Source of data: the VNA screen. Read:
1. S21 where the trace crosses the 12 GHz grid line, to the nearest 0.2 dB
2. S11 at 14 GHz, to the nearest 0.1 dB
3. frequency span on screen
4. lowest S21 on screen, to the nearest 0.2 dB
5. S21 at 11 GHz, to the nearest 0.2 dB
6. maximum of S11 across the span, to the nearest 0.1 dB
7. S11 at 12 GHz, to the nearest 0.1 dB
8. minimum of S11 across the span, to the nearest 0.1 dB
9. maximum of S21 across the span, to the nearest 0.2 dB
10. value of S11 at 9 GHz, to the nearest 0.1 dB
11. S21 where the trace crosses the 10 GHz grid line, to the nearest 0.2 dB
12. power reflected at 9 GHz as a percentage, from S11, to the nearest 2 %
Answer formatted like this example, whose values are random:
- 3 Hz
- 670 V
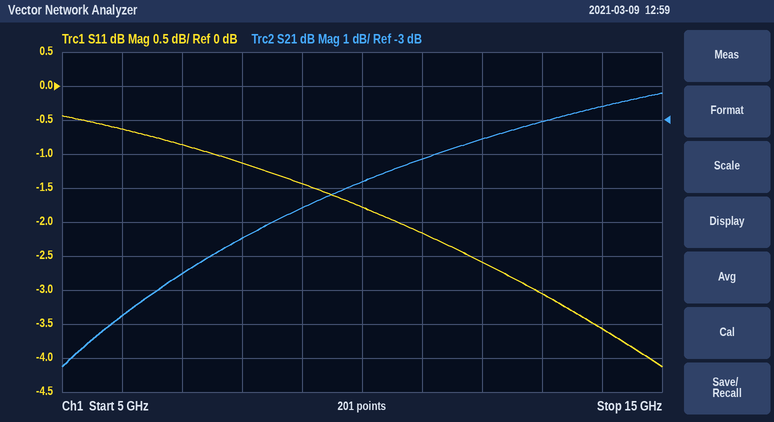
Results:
- -3.6 dB
- -3.6 dB
- 10 GHz
- -10.2 dB
- -4.2 dB
- -0.4 dB
- -2.6 dB
- -4.1 dB
- -2.2 dB
- -1.4 dB
- -4.8 dB
- 72 %
